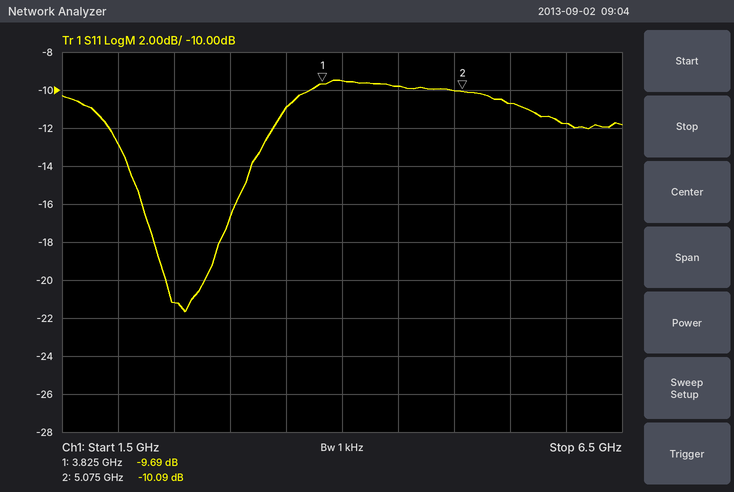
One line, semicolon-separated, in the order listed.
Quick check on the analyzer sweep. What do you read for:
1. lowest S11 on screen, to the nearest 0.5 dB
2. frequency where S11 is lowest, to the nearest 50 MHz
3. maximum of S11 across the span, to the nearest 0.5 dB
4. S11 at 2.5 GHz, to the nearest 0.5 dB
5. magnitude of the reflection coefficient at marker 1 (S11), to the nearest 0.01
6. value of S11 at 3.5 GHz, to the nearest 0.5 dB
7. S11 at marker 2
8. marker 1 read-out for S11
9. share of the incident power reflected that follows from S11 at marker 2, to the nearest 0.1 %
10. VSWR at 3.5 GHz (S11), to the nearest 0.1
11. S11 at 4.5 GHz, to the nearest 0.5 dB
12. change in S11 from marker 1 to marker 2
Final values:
-21.5 dB; 2.60 GHz; -9.5 dB; -21.0 dB; 0.33; -11.0 dB; -10.09 dB; -9.69 dB; 9.8 %; 1.8; -10.0 dB; -0.40 dB
